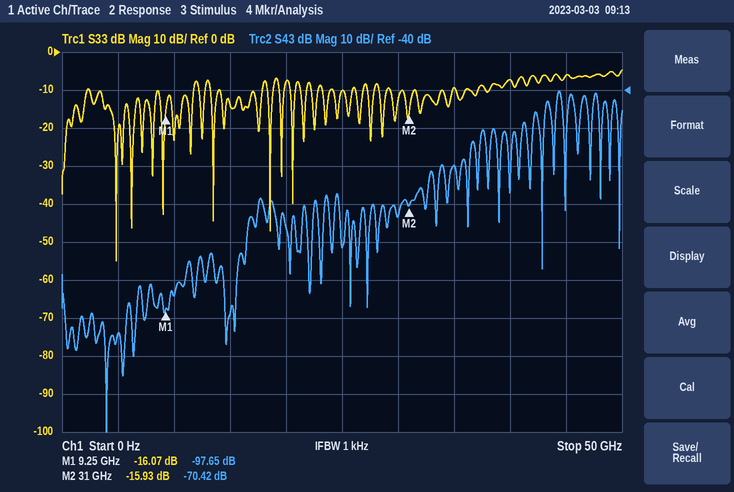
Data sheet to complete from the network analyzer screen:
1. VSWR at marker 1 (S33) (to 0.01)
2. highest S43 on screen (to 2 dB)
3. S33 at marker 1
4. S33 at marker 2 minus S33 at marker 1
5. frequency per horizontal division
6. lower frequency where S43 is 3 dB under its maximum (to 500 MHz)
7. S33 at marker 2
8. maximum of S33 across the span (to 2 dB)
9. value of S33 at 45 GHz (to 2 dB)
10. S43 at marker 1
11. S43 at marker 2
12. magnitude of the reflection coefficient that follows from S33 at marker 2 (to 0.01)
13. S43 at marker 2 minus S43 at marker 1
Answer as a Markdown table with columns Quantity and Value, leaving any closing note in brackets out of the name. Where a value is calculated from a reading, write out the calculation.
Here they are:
| Quantity | Value |
|---|---|
| VSWR at marker 1 (S33) | (1 + 0.1572)/(1 − 0.1572) ≈ 1.37 |
| highest S43 on screen | -40 dB |
| S33 at marker 1 | -16.07 dB |
| S33 at marker 2 minus S33 at marker 1 | -15.93 − (-16.07) = 0.14 dB |
| frequency per horizontal division | 5 GHz |
| lower frequency where S43 is 3 dB under its maximum | 44.0 GHz |
| S33 at marker 2 | -15.93 dB |
| maximum of S33 across the span | -4 dB |
| value of S33 at 45 GHz | -6 dB |
| S43 at marker 1 | -97.65 dB |
| S43 at marker 2 | -70.42 dB |
| magnitude of the reflection coefficient that follows from S33 at marker 2 | 10^(-15.93/20) ≈ 0.16 |
| S43 at marker 2 minus S43 at marker 1 | -70.42 − (-97.65) = 27.23 dB |
